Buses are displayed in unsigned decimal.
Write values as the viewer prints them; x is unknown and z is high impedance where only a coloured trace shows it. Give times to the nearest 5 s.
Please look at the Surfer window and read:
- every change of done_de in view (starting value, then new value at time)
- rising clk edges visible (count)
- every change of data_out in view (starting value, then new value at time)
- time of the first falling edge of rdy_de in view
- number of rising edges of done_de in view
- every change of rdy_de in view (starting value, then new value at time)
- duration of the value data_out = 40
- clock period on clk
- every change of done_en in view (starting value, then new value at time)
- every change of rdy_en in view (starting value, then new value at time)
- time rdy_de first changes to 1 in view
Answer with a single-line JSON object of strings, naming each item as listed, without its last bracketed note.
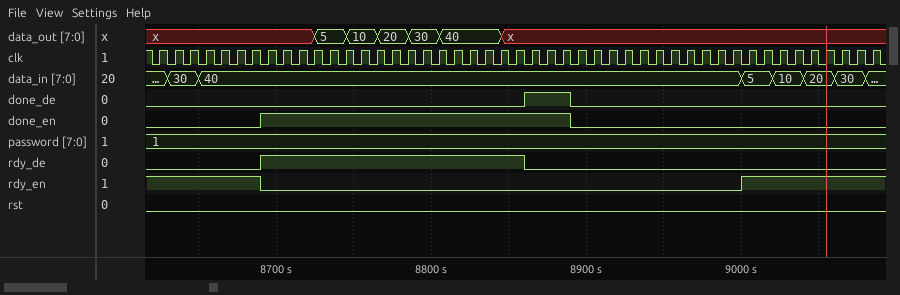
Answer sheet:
{"every change of done_de in view": "0, 1 at 8860 s, 0 at 8890 s", "rising clk edges visible": "47", "every change of data_out in view": "x, 5 at 8725 s, 10 at 8745 s, 20 at 8765 s, 30 at 8785 s, 40 at 8805 s, x at 8845 s", "time of the first falling edge of rdy_de in view": "8860 s", "number of rising edges of done_de in view": "1", "every change of rdy_de in view": "0, 1 at 8690 s, 0 at 8860 s", "duration of the value data_out = 40": "40 s", "clock period on clk": "10 s", "every change of done_en in view": "0, 1 at 8690 s, 0 at 8890 s", "every change of rdy_en in view": "1, 0 at 8690 s, 1 at 9000 s", "time rdy_de first changes to 1 in view": "8690 s"}
